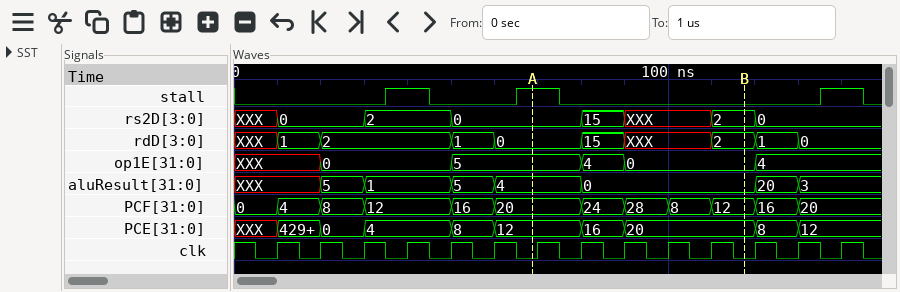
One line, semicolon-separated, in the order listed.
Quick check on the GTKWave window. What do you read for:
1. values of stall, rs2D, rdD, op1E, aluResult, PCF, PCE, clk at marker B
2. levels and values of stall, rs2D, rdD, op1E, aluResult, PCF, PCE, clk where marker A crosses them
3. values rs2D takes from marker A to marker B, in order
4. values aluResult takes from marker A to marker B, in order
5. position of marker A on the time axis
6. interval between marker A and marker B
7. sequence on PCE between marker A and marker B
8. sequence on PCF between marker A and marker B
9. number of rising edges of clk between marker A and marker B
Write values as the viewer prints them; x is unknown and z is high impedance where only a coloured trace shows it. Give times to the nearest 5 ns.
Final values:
stall=0, rs2D=2, rdD=2, op1E=0, aluResult=0, PCF=12, PCE=20, clk=0; stall=1, rs2D=0, rdD=0, op1E=5, aluResult=4, PCF=20, PCE=12, clk=0; 0, 15, XXX, 2; 4, 0; 70 ns; 50 ns; 12, 16, 20; 20, 24, 28, 8, 12; 5
